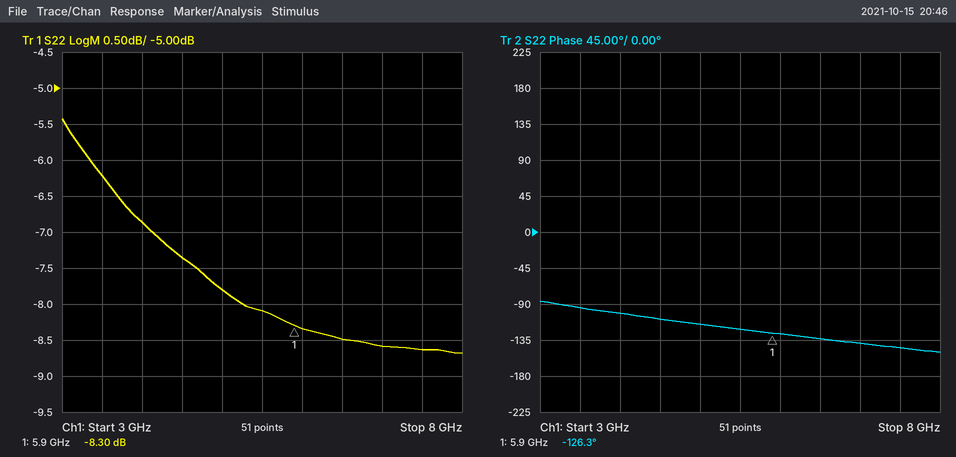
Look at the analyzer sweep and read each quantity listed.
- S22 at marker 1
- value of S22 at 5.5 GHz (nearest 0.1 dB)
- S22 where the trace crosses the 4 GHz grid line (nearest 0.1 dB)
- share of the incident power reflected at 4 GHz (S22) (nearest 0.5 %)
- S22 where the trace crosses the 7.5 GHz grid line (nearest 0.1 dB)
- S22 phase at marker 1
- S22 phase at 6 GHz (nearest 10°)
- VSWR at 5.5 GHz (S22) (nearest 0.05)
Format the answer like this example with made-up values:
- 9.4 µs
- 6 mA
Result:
- -8.30 dB
- -8.1 dB
- -6.9 dB
- 20.5 %
- -8.6 dB
- -126.3°
- -130°
- 2.30
